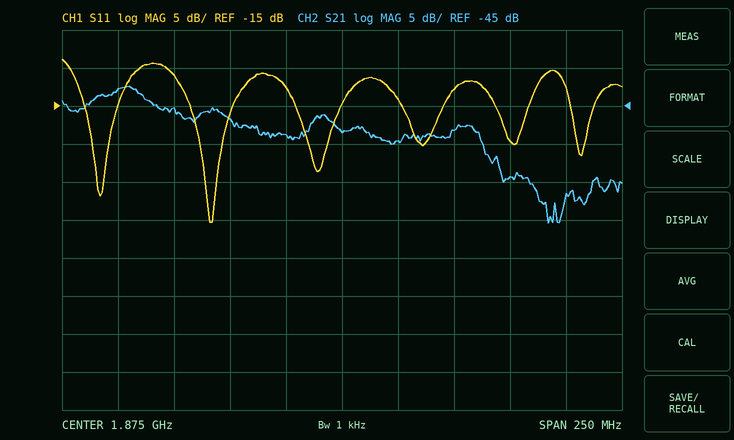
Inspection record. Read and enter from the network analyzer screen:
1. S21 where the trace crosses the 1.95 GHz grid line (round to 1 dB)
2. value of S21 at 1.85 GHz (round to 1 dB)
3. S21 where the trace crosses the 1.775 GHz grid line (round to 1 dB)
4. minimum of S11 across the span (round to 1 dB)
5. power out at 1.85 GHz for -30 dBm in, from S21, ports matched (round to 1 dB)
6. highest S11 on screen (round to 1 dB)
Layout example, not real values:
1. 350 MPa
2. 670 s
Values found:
1. -54 dB
2. -49 dB
3. -43 dB
4. -30 dB
5. -79 dBm
6. -9 dB
